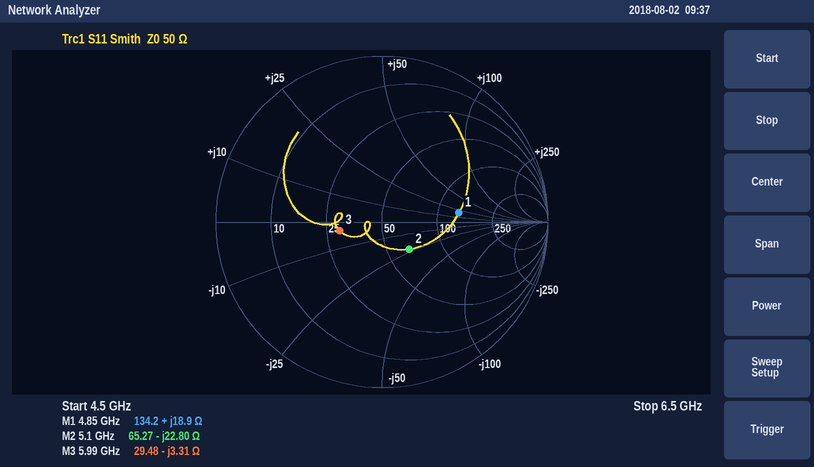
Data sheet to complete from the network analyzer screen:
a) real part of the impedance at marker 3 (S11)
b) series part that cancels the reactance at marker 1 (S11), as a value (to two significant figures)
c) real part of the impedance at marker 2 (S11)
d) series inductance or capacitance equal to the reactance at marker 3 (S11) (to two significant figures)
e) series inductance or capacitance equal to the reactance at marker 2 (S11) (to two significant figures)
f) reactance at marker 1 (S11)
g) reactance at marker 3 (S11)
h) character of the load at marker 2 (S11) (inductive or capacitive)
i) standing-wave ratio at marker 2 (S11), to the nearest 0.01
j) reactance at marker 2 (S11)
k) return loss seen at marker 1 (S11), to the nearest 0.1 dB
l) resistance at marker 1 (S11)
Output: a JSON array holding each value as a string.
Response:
["29.48 Ω", "1.7 pF", "65.27 Ω", "8.0 pF", "1.4 pF", "+18.9 Ω", "-3.31 Ω", "capacitive", "1.61", "-22.80 Ω", "6.6 dB", "134.2 Ω"]
